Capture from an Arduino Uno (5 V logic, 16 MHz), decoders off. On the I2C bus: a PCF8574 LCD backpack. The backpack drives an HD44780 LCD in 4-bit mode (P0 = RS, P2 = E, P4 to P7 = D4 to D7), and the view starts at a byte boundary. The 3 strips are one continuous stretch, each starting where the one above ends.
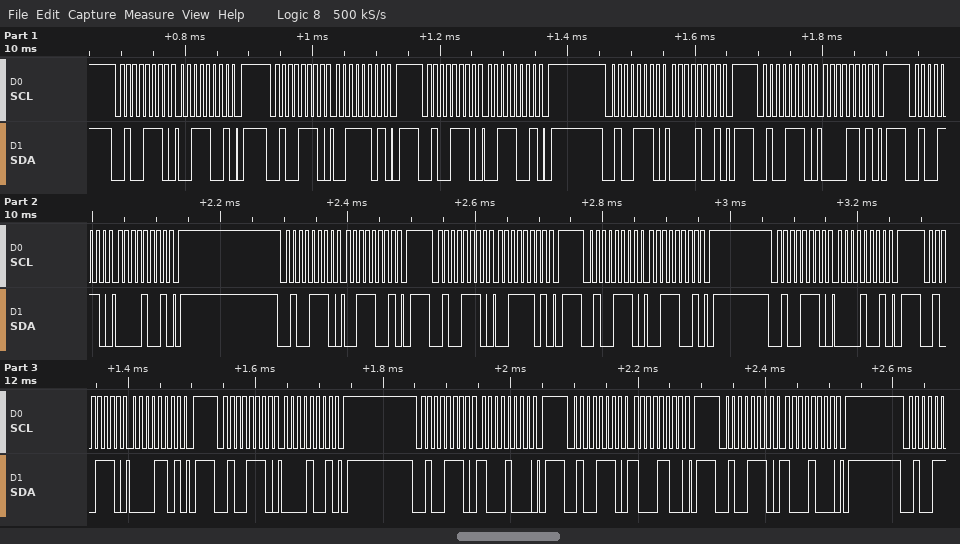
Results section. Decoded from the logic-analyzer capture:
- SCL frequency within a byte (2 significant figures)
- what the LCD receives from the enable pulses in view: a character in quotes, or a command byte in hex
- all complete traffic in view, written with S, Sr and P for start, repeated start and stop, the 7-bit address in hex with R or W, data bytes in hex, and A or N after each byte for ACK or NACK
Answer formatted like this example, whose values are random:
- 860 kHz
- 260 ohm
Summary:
- 100 kHz
- '0' '0'
- S 27W A 39 A P S 27W A 3D A P S 27W A 39 A P S 27W A 09 A P S 27W A 0D A P S 27W A 09 A P S 27W A 39 A P S 27W A 3D A P S 27W A 39 A P S 27W A 09 A P S 27W A 0D A P S 27W A 09 A P S 27W A 88 A P S 27W A 8C A P S 27W A 88 A P
